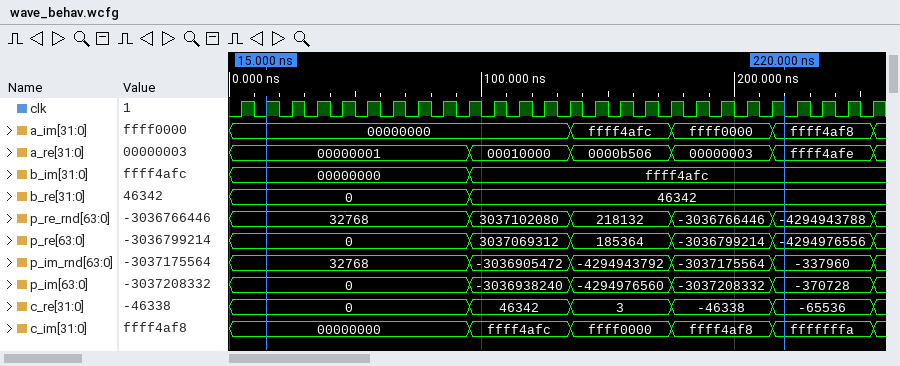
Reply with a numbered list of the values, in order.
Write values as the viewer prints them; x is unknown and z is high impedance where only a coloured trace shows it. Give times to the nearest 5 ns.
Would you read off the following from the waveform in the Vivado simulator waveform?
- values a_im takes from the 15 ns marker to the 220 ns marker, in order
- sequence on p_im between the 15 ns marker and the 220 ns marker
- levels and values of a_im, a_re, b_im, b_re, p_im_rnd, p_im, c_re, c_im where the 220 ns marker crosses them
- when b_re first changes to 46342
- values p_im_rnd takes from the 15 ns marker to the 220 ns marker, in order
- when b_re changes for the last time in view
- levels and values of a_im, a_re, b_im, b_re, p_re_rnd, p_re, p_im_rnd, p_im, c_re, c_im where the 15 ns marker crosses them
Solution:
1. 00000000, ffff4afc, ffff0000, ffff4af8
2. 0, -3036938240, -4294976560, -3037208332, -370728
3. a_im=ffff4af8, a_re=ffff4afe, b_im=ffff4afc, b_re=46342, p_im_rnd=-337960, p_im=-370728, c_re=-65536, c_im=fffffffa
4. 95 ns
5. 32768, -3036905472, -4294943792, -3037175564, -337960
6. 95 ns
7. a_im=00000000, a_re=00000001, b_im=00000000, b_re=0, p_re_rnd=32768, p_re=0, p_im_rnd=32768, p_im=0, c_re=0, c_im=00000000
